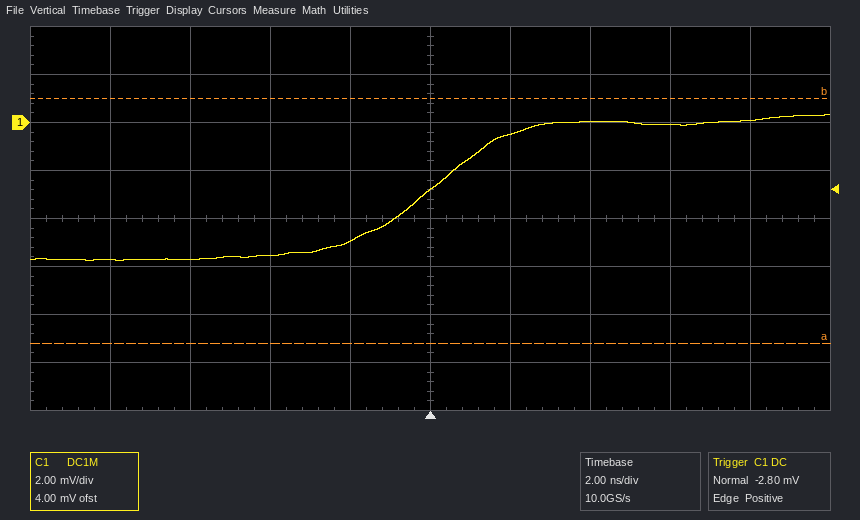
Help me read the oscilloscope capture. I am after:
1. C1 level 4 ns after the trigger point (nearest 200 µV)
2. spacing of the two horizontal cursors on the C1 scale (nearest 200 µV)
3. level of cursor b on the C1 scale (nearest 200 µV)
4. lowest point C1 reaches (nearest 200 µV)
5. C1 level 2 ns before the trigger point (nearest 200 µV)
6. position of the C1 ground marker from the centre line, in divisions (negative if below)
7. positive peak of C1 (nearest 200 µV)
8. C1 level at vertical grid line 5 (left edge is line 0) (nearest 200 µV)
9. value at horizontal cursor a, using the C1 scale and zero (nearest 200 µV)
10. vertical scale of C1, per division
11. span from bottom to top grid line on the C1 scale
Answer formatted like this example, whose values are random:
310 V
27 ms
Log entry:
0.0 mV
10.2 mV
1.0 mV
-5.8 mV
-5.0 mV
+2.0 div
400 µV
-2.8 mV
-9.2 mV
2 mV
16 mV
